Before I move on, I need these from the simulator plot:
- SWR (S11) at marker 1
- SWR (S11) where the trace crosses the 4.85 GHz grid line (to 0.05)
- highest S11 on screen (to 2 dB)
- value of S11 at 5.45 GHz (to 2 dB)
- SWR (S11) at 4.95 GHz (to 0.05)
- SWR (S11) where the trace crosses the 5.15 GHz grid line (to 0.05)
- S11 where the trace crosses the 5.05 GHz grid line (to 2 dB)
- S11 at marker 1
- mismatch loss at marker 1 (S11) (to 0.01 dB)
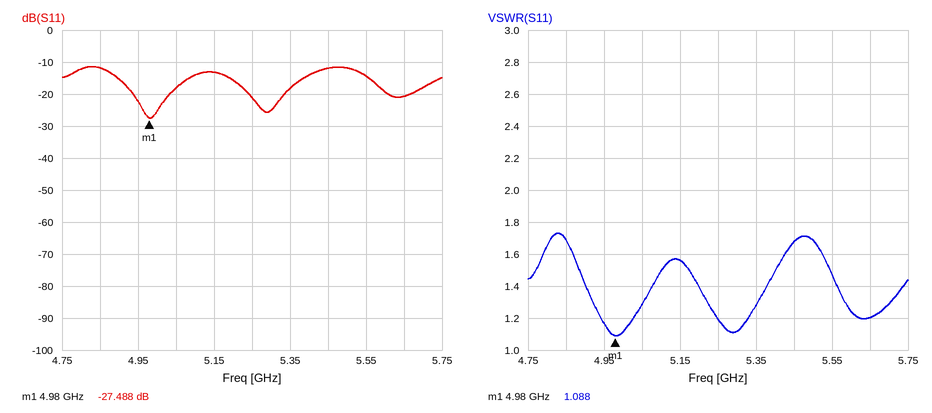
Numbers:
1.088
1.70
-12 dB
-12 dB
1.15
1.55
-18 dB
-27.488 dB
0.01 dB
